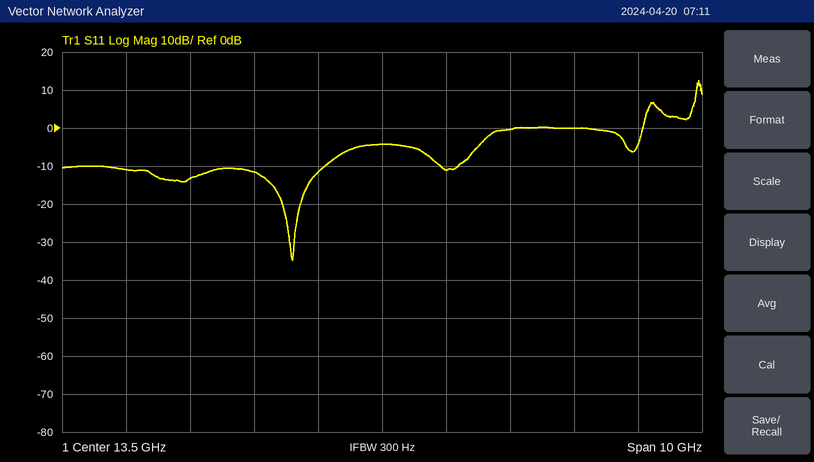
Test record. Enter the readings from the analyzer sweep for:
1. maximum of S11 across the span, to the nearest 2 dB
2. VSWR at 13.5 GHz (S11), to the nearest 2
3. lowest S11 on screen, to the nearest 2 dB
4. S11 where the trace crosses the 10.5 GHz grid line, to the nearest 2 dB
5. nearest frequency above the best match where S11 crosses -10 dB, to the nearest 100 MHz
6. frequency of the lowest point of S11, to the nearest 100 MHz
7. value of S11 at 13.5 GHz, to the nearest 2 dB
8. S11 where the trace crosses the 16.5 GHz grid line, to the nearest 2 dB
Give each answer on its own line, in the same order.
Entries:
12 dB
4
-34 dB
-14 dB
12.6 GHz
12.1 GHz
-4 dB
0 dB
